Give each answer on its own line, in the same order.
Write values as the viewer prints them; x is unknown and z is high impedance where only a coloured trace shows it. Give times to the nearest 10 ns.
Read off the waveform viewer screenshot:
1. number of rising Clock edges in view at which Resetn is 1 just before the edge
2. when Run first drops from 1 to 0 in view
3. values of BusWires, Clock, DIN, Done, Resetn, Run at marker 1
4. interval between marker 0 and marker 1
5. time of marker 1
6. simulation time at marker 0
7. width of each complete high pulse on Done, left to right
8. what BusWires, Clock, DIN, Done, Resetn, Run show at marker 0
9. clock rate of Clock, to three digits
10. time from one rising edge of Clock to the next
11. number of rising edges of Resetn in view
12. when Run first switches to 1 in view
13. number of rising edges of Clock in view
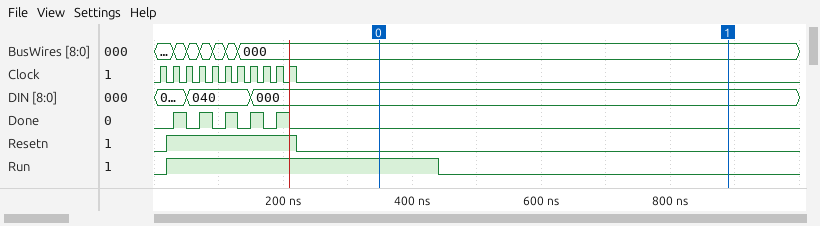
10
440 ns
BusWires=000, Clock=0, DIN=000, Done=0, Resetn=0, Run=0
540 ns
890 ns
350 ns
20 ns, 20 ns, 20 ns, 20 ns, 20 ns
BusWires=000, Clock=0, DIN=000, Done=0, Resetn=0, Run=1
50.0 MHz
20 ns
1
20 ns
11
